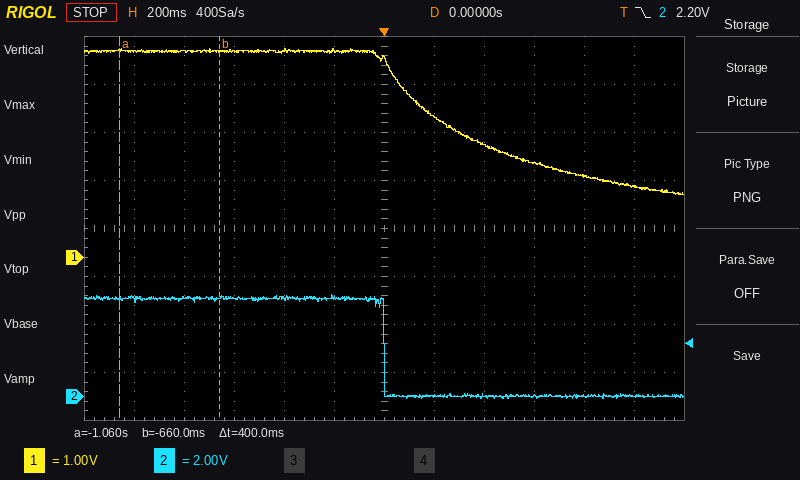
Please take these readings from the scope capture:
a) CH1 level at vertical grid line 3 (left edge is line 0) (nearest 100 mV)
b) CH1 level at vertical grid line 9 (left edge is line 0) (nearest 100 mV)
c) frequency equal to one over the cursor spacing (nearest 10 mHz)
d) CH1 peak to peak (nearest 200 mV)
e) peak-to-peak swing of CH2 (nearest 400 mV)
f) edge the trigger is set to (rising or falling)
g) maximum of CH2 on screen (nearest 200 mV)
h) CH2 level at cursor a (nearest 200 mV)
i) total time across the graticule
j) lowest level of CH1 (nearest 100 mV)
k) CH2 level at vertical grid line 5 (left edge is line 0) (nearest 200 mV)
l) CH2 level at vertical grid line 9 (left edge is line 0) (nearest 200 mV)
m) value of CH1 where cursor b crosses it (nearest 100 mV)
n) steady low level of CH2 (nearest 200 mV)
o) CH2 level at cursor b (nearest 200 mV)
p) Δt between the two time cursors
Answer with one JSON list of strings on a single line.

["4.3 V", "2.0 V", "2.50 Hz", "3.0 V", "4.4 V", "falling", "4.2 V", "4.0 V", "2.4 s", "1.3 V", "4.2 V", "0.0 V", "4.3 V", "0.0 V", "4.2 V", "400 ms"]
